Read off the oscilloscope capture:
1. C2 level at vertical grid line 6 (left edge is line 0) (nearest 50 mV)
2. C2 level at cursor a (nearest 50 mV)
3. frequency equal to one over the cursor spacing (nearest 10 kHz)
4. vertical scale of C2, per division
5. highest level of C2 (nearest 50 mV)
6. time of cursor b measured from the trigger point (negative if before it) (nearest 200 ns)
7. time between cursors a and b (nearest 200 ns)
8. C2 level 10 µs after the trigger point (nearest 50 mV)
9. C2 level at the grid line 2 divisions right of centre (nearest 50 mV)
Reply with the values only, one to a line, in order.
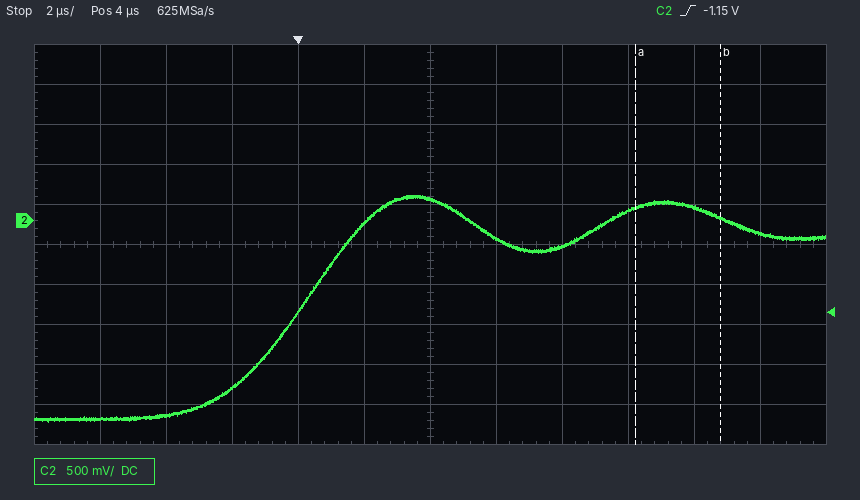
250 mV
150 mV
380 kHz
500 mV
300 mV
+12.8 µs
2.6 µs
100 mV
-350 mV
